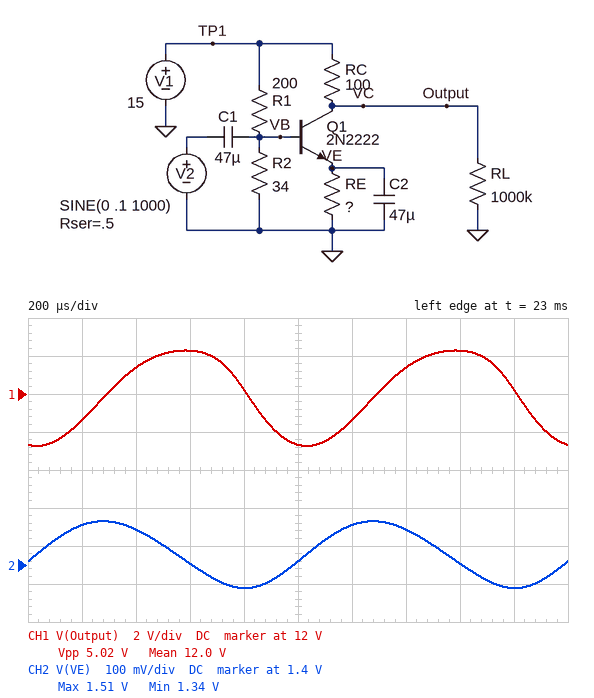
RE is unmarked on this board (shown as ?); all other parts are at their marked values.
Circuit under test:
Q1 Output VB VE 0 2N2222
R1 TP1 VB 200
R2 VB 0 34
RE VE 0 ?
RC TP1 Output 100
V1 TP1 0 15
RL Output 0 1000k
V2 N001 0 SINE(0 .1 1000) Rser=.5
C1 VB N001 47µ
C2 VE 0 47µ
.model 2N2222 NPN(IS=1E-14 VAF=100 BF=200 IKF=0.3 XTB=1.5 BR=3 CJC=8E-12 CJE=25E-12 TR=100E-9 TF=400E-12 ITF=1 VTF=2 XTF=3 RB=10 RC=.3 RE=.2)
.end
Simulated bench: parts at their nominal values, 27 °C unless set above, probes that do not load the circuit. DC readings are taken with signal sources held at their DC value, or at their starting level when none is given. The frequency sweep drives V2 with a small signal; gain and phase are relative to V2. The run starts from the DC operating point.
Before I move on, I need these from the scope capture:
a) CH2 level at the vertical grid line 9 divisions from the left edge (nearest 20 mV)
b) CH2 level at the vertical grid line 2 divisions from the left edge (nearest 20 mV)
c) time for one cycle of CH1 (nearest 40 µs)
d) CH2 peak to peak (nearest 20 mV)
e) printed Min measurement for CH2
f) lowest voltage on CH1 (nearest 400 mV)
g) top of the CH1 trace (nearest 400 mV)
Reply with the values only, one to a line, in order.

1.34 V
1.50 V
1.00 ms
180 mV
1.34 V
9.2 V
14.4 V
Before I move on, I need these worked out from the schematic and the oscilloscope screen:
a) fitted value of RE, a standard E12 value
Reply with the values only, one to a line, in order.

47 Ω
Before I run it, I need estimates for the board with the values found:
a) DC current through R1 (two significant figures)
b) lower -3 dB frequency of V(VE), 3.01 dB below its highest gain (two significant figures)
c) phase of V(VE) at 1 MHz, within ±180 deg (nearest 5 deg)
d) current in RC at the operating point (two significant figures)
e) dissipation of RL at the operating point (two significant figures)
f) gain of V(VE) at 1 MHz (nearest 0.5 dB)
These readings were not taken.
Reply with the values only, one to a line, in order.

64 mA
110 Hz
-90 deg
30 mA
140 µW
-51.0 dB
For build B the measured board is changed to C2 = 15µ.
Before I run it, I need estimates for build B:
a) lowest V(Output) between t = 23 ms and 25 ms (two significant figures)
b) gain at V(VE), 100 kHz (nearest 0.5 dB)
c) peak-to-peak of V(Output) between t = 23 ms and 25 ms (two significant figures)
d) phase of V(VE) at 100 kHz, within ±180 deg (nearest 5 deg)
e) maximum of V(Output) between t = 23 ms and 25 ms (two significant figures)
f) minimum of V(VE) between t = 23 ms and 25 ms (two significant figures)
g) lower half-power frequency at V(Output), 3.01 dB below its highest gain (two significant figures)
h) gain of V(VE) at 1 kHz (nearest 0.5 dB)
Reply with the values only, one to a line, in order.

11 V
-21.5 dB
1.8 V
-85 deg
13 V
1.3 V
9.0 kHz
-0.5 dB
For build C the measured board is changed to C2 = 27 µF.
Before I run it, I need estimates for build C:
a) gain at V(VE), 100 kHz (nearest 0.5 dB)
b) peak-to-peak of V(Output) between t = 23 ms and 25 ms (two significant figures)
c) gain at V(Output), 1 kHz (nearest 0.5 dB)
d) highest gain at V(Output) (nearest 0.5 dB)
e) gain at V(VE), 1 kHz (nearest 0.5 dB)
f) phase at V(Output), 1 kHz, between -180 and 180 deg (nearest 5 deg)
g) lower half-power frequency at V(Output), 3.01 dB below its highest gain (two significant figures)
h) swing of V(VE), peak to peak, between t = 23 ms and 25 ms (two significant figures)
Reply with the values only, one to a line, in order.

-26.5 dB
3.1 V
24.0 dB
38.0 dB
-0.5 dB
-100 deg
5.0 kHz
190 mV
